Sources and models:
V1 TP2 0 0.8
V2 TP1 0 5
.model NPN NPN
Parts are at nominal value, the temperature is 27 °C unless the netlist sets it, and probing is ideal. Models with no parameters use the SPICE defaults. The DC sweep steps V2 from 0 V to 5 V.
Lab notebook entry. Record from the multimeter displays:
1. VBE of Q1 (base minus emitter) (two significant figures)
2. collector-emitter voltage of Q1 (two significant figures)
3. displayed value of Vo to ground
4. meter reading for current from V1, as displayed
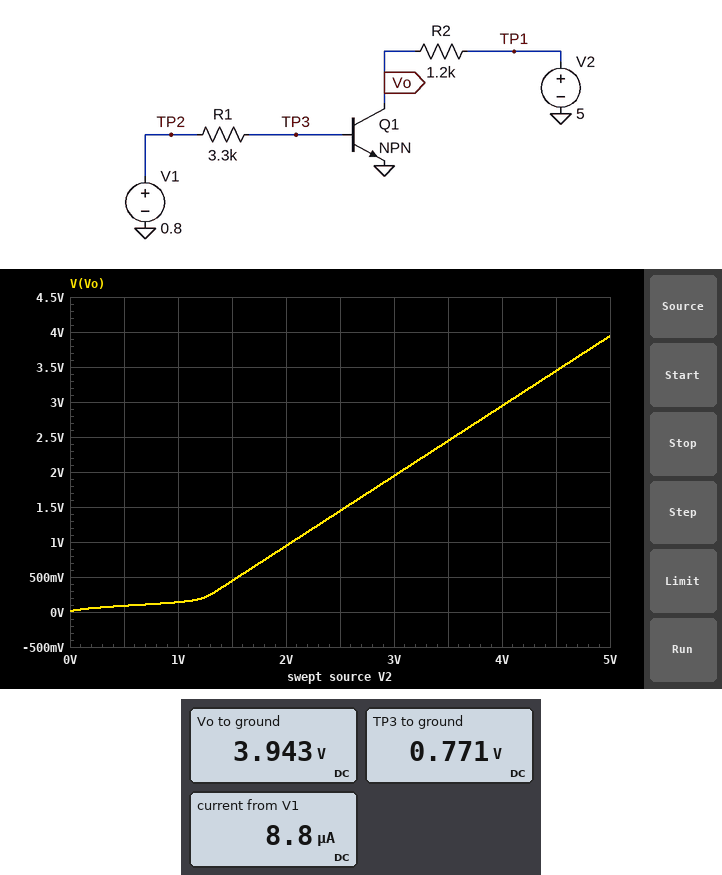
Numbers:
770 mV
3.9 V
3.943 V
8.8 µA
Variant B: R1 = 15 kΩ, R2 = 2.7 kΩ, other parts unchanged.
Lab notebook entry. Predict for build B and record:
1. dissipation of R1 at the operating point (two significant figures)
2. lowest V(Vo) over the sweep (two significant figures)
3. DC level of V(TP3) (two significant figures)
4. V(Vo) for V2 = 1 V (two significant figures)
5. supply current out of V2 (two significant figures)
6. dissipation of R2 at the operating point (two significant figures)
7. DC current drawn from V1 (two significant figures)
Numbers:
190 nW
11 mV
750 mV
160 mV
350 µA
330 µW
3.5 µA
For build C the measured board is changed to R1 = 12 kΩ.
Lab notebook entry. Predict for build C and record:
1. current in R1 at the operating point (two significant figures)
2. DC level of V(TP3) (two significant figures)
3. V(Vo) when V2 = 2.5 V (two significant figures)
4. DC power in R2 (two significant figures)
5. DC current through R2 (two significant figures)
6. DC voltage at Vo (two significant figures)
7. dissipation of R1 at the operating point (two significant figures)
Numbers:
4.1 µA
750 mV
2.0 V
200 µW
410 µA
4.5 V
200 nW
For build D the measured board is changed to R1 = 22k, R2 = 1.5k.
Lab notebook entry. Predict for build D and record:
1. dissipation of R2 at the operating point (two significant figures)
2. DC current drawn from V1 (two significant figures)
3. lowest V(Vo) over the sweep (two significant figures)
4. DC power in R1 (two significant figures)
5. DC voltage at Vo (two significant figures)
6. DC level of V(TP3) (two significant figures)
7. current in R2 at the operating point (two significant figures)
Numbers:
110 µW
2.7 µA
6.9 mV
160 nW
4.6 V
740 mV
270 µA
